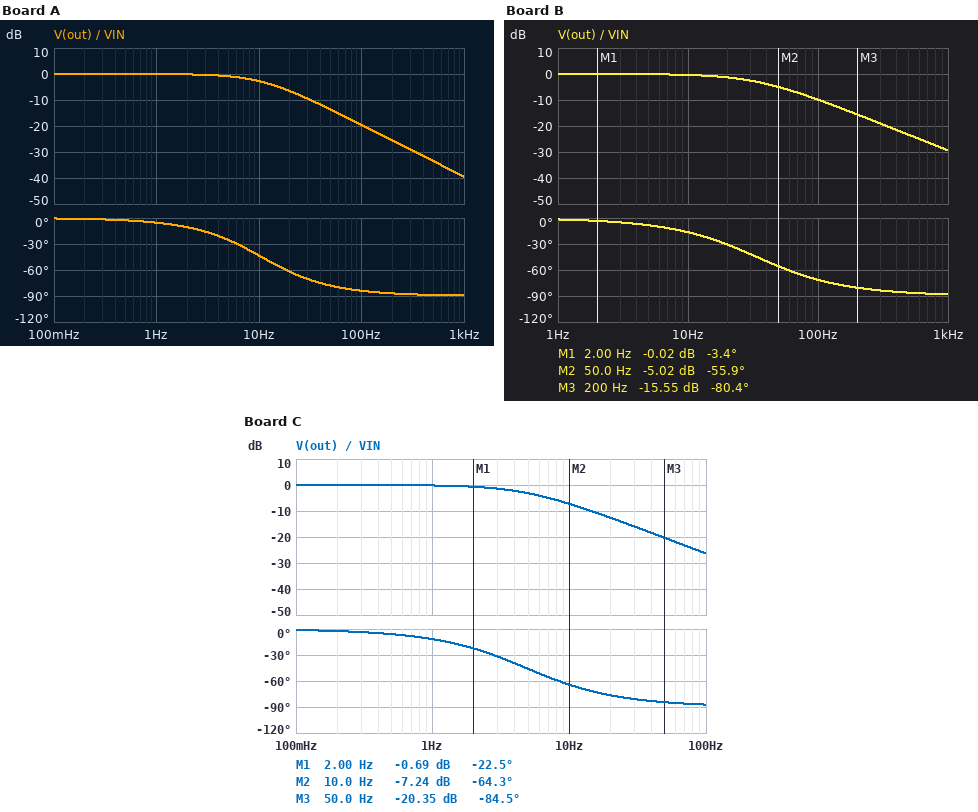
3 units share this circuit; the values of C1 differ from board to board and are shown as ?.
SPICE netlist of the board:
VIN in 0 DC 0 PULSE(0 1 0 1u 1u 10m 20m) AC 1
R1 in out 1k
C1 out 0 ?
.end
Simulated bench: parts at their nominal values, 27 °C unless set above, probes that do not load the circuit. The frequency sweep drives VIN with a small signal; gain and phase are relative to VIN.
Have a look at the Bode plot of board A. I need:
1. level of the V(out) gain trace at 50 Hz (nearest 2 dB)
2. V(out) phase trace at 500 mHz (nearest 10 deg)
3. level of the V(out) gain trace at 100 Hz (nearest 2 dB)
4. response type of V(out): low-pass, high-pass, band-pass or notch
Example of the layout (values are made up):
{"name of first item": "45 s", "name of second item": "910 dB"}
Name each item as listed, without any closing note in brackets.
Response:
{"level of the V(out) gain trace at 50 Hz": "-14 dB", "V(out) phase trace at 500 mHz": "0 deg", "level of the V(out) gain trace at 100 Hz": "-20 dB", "response type of V(out): low-pass, high-pass, band-pass or notch": "low-pass"}
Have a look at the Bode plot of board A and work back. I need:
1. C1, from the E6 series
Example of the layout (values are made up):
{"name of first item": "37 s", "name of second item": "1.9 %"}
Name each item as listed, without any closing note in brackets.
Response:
{"C1, from the E6 series": "15 µF"}
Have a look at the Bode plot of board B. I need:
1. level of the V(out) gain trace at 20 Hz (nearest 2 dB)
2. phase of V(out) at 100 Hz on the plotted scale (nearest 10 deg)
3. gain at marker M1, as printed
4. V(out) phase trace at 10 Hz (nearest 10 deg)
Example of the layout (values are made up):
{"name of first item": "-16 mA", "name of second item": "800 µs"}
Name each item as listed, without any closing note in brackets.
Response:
{"level of the V(out) gain trace at 20 Hz": "-2 dB", "phase of V(out) at 100 Hz on the plotted scale": "-70 deg", "gain at marker M1, as printed": "-0.02 dB", "V(out) phase trace at 10 Hz": "-20 deg"}
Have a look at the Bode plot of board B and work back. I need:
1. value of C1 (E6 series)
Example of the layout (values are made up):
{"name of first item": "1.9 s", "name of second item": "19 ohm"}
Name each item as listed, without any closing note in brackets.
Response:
{"value of C1": "4.7 µF"}
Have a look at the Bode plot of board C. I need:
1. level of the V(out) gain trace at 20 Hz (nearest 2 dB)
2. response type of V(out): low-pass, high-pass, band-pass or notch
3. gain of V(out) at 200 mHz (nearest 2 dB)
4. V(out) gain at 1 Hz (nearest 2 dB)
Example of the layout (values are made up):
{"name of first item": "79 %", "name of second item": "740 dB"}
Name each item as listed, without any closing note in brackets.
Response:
{"level of the V(out) gain trace at 20 Hz": "-12 dB", "response type of V(out): low-pass, high-pass, band-pass or notch": "low-pass", "gain of V(out) at 200 mHz": "0 dB", "V(out) gain at 1 Hz": "0 dB"}
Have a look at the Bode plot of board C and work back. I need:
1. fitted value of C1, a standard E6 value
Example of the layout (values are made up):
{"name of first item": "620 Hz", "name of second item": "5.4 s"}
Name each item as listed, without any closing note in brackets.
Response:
{"fitted value of C1, a standard E6 value": "33 µF"}
